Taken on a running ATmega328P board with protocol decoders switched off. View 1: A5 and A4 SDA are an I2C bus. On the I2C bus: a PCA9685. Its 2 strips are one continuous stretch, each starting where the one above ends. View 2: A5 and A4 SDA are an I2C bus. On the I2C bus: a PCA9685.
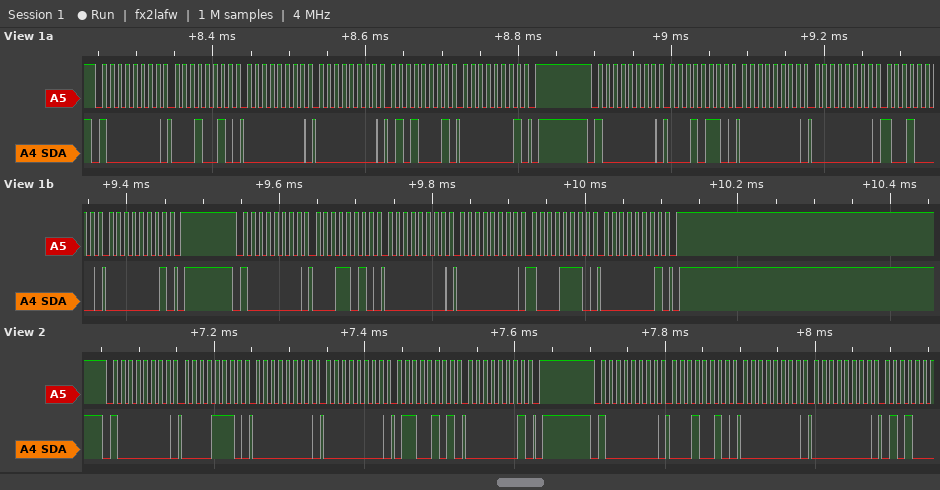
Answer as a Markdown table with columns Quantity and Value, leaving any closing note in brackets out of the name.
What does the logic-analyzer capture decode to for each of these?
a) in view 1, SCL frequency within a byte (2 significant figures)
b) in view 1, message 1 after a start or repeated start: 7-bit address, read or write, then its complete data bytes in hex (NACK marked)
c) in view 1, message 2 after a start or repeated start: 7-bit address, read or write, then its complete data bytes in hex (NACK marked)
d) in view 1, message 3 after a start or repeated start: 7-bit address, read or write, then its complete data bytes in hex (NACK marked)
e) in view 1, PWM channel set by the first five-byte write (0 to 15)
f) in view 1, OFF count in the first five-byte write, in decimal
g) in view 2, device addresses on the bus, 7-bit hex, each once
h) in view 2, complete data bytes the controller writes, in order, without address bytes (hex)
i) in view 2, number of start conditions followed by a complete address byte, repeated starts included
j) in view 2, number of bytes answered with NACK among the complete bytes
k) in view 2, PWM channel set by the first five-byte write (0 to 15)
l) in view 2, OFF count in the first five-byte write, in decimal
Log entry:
| Quantity | Value |
|---|---|
| in view 1, SCL frequency within a byte | 100 kHz |
| in view 1, message 1 after a start or repeated start: 7-bit address, read or write, then its complete data bytes in hex | 0x40 write: 12 00 00 51 01 |
| in view 1, message 2 after a start or repeated start: 7-bit address, read or write, then its complete data bytes in hex | 0x40 write: 16 00 00 90 01 |
| in view 1, message 3 after a start or repeated start: 7-bit address, read or write, then its complete data bytes in hex | 0x40 write: 1A 00 00 8E 01 |
| in view 1, PWM channel set by the first five-byte write | 3 |
| in view 1, OFF count in the first five-byte write, in decimal | 337 |
| in view 2, device addresses on the bus, 7-bit hex, each once | 0x40 |
| in view 2, complete data bytes the controller writes, in order, without address bytes | 0E 00 00 65 01 12 00 00 |
| in view 2, number of start conditions followed by a complete address byte, repeated starts included | 2 |
| in view 2, number of bytes answered with NACK among the complete bytes | 0 |
| in view 2, PWM channel set by the first five-byte write | 2 |
| in view 2, OFF count in the first five-byte write, in decimal | 357 |
